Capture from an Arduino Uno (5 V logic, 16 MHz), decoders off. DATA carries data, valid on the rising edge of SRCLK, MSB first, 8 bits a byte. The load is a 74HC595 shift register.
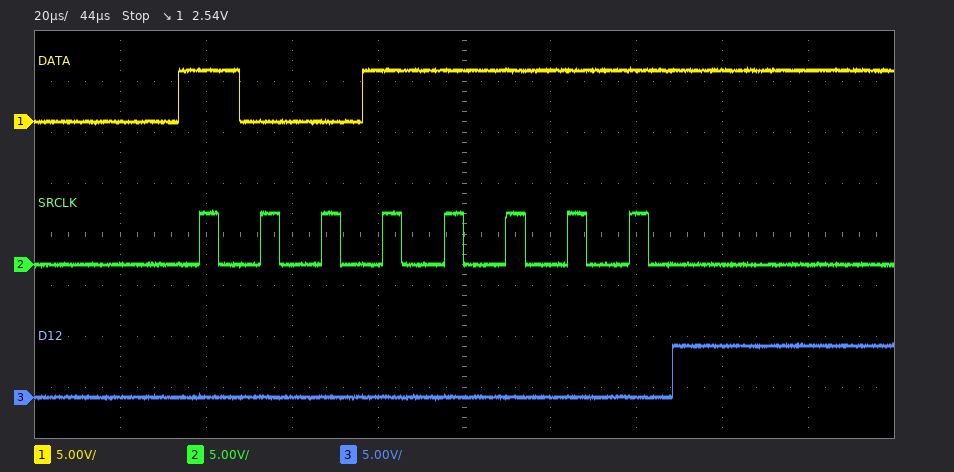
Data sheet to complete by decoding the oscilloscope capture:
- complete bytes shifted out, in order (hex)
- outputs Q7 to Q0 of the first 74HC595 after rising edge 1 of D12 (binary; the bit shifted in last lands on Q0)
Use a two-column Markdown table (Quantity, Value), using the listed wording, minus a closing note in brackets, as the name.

| Quantity | Value |
|---|---|
| complete bytes shifted out, in order | 9F |
| outputs Q7 to Q0 of the first 74HC595 after rising edge 1 of D12 | 10011111 |
